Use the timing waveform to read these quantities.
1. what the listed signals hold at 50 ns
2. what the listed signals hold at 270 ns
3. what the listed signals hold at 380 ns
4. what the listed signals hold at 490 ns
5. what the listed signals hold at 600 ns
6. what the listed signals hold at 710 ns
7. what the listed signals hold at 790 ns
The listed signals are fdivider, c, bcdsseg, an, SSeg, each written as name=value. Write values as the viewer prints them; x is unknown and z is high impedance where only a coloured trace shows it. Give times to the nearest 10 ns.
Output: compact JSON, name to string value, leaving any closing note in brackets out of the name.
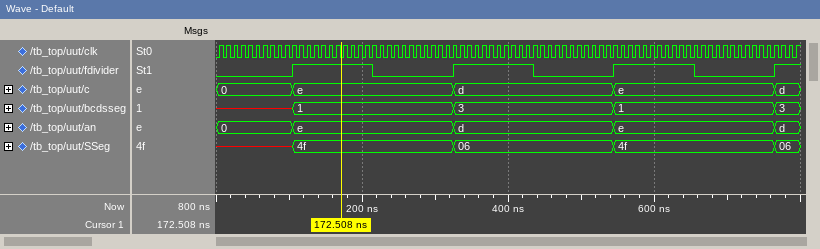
{"what the listed signals hold at 50 ns": "fdivider=0, c=0, bcdsseg=x, an=0, SSeg=x", "what the listed signals hold at 270 ns": "fdivider=0, c=e, bcdsseg=1, an=e, SSeg=4f", "what the listed signals hold at 380 ns": "fdivider=1, c=d, bcdsseg=3, an=d, SSeg=06", "what the listed signals hold at 490 ns": "fdivider=0, c=d, bcdsseg=3, an=d, SSeg=06", "what the listed signals hold at 600 ns": "fdivider=1, c=e, bcdsseg=1, an=e, SSeg=4f", "what the listed signals hold at 710 ns": "fdivider=0, c=e, bcdsseg=1, an=e, SSeg=4f", "what the listed signals hold at 790 ns": "fdivider=1, c=d, bcdsseg=3, an=d, SSeg=06"}
